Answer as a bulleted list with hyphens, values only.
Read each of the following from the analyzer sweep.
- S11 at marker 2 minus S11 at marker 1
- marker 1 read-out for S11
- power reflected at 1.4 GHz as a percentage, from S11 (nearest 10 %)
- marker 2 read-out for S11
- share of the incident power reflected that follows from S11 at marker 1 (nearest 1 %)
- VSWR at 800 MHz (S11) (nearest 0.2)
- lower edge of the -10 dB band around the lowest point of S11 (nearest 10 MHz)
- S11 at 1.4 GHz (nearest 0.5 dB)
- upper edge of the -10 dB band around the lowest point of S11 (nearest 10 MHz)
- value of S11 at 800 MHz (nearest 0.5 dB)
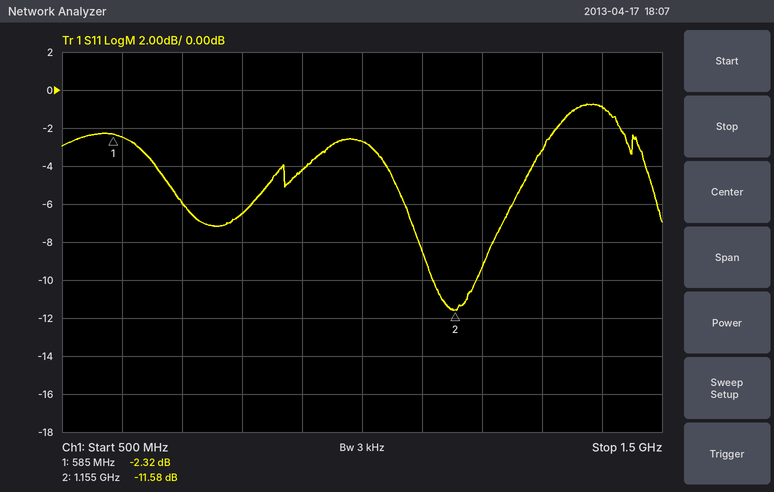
- -9.26 dB
- -2.32 dB
- 80 %
- -11.58 dB
- 59 %
- 2.8
- 1.12 GHz
- -1.0 dB
- 1.19 GHz
- -6.5 dB
